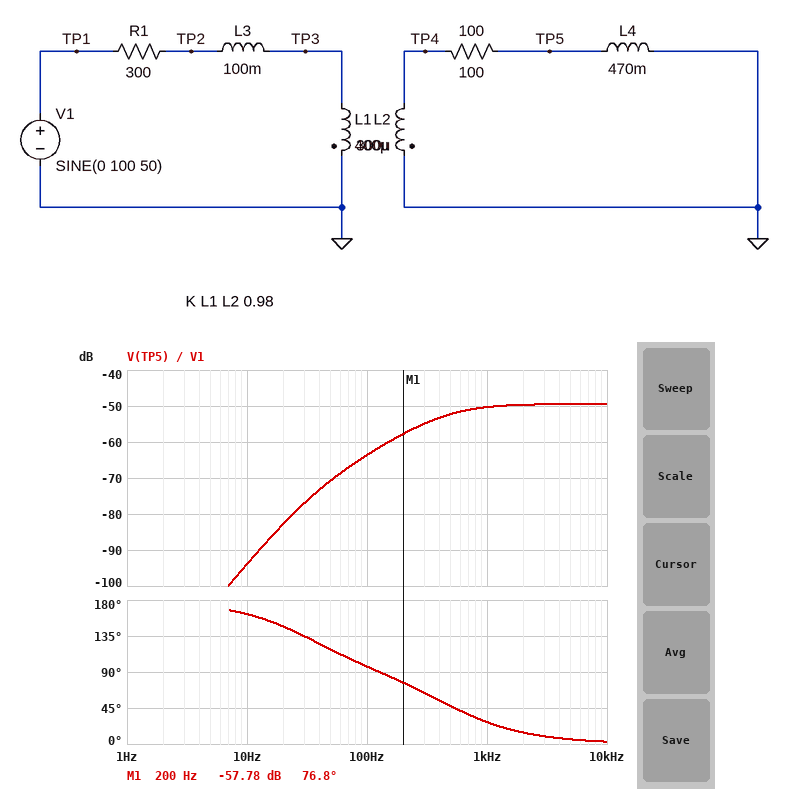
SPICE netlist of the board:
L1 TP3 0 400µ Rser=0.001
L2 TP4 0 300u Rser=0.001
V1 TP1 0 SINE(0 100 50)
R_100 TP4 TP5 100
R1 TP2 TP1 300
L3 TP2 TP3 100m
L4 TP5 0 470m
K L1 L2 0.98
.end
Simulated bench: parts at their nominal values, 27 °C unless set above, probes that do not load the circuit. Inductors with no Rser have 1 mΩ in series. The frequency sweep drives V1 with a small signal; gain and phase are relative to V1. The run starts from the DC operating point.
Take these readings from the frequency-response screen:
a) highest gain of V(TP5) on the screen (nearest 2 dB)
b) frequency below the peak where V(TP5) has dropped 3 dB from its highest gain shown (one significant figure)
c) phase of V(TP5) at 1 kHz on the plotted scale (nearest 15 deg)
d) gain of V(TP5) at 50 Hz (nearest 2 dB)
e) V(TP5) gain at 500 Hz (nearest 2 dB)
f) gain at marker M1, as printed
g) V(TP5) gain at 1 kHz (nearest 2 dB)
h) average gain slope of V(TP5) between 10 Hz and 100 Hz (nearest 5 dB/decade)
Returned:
-50 dB
500 Hz
30 deg
-70 dB
-52 dB
-57.78 dB
-50 dB
30 dB/decade
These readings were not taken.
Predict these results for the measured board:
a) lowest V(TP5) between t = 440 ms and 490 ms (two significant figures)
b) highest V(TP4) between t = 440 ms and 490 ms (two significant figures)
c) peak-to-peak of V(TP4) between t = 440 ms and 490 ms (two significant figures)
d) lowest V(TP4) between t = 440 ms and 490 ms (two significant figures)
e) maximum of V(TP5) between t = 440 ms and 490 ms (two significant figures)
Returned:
-29 mV
35 mV
71 mV
-35 mV
29 mV
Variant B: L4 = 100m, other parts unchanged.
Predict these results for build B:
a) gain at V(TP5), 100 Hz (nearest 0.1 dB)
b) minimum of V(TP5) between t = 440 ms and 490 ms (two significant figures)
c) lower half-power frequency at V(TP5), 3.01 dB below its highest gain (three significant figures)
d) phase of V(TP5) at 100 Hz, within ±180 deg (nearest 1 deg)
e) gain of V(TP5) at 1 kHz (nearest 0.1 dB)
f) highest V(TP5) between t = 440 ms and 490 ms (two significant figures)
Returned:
-68.6 dB
-11 mV
522 Hz
136 deg
-50.4 dB
11 mV
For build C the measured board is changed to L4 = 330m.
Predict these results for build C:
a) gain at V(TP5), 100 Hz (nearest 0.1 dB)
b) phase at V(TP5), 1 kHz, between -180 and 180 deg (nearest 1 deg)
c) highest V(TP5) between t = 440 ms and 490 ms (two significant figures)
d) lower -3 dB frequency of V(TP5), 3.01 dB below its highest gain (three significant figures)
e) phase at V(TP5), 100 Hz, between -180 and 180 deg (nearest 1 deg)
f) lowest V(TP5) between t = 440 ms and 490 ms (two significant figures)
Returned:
-64.1 dB
28 deg
25 mV
480 Hz
104 deg
-25 mV
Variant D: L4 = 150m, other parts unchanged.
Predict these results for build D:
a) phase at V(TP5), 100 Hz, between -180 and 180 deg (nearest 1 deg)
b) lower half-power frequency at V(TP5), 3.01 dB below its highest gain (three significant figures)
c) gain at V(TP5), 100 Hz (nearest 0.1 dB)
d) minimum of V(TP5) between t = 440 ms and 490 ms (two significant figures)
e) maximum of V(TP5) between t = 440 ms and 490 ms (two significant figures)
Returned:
125 deg
498 Hz
-66.4 dB
-15 mV
15 mV
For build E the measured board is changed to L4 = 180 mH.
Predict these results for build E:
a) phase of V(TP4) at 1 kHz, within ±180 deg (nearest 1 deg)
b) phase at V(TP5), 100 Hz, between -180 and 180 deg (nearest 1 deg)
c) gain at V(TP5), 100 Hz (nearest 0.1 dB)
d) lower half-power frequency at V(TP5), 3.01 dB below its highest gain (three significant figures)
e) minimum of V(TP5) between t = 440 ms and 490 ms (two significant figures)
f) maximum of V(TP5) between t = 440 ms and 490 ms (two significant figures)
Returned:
25 deg
120 deg
-65.7 dB
491 Hz
-17 mV
17 mV
